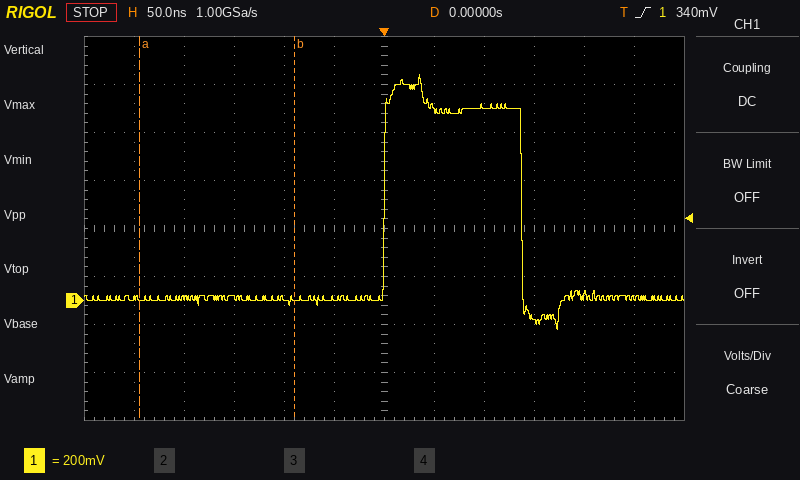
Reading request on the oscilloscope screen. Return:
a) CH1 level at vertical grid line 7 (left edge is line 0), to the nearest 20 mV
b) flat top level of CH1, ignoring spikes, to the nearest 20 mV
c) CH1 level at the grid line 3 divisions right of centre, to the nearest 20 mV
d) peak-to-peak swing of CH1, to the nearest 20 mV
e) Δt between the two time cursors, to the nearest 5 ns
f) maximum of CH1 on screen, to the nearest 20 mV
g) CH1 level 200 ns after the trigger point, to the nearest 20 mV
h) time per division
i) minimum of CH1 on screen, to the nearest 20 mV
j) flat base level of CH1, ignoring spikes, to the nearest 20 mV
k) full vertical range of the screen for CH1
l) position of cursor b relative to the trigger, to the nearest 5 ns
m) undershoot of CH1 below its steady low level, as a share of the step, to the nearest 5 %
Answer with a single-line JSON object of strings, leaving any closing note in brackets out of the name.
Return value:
{"CH1 level at vertical grid line 7 (left edge is line 0), to the nearest 20 mV": "800 mV", "flat top level of CH1, ignoring spikes, to the nearest 20 mV": "800 mV", "CH1 level at the grid line 3 divisions right of centre, to the nearest 20 mV": "-80 mV", "peak-to-peak swing of CH1, to the nearest 20 mV": "1.06 V", "Δt between the two time cursors, to the nearest 5 ns": "155 ns", "maximum of CH1 on screen, to the nearest 20 mV": "940 mV", "CH1 level 200 ns after the trigger point, to the nearest 20 mV": "20 mV", "time per division": "50 ns", "minimum of CH1 on screen, to the nearest 20 mV": "-120 mV", "flat base level of CH1, ignoring spikes, to the nearest 20 mV": "0 mV", "full vertical range of the screen for CH1": "1.6 V", "position of cursor b relative to the trigger, to the nearest 5 ns": "-90 ns", "undershoot of CH1 below its steady low level, as a share of the step, to the nearest 5 %": "15 %"}
